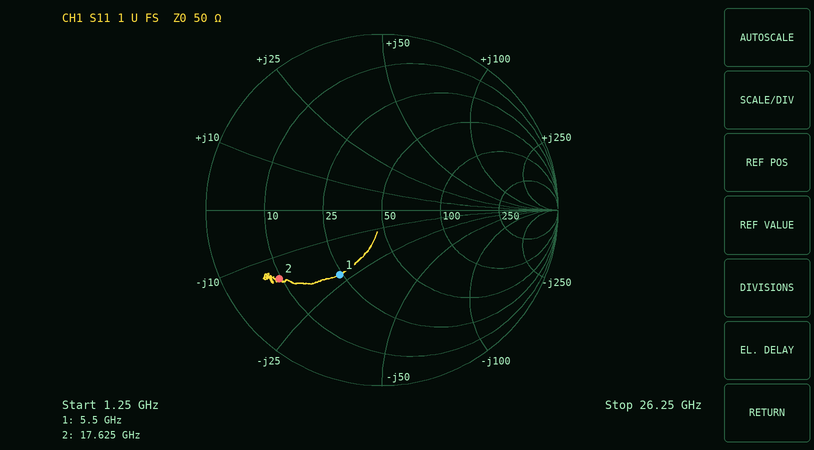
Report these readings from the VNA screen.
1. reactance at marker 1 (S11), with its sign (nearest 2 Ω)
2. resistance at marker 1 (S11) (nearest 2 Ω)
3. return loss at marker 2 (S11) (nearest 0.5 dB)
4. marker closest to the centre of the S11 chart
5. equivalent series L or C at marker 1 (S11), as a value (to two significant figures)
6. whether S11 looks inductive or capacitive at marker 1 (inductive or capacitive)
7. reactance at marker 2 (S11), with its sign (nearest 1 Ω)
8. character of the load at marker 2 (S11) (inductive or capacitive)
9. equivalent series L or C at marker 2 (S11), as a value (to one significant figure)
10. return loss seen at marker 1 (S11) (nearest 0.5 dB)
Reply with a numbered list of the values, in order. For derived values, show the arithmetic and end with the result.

1. -22 Ω
2. 24 Ω
3. 3.0 dB
4. marker 1
5. C = 1/(2π × 5.5 GHz × 22 Ω) ≈ 1.3 pF
6. capacitive
7. -15 Ω
8. capacitive
9. C = 1/(2π × 17.625 GHz × 15 Ω) ≈ 602 fF, so 600 fF to one significant figure
10. 7.0 dB
